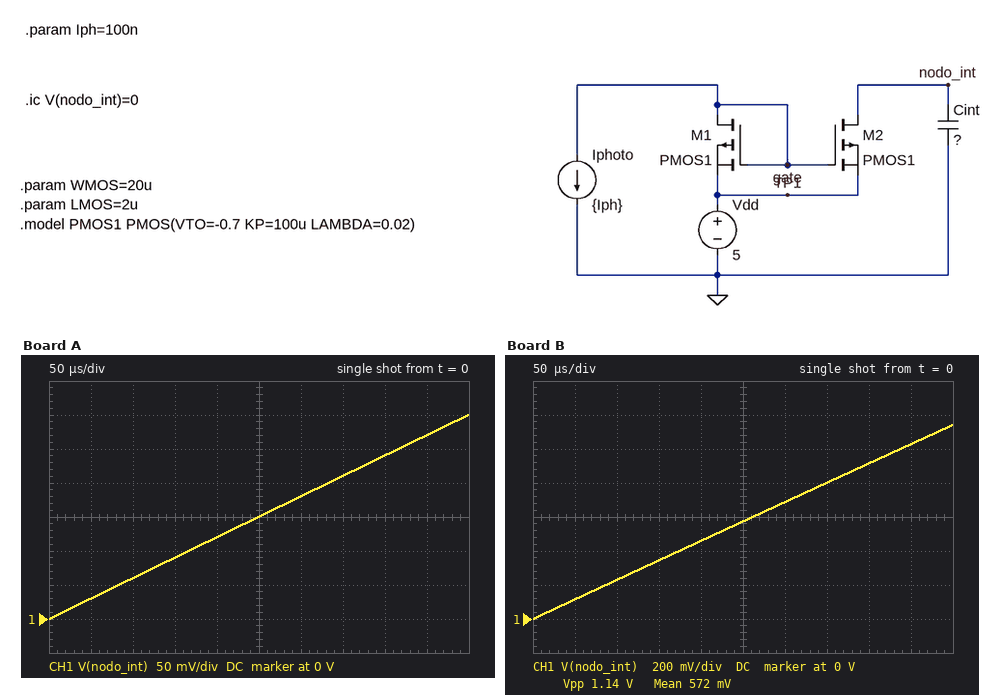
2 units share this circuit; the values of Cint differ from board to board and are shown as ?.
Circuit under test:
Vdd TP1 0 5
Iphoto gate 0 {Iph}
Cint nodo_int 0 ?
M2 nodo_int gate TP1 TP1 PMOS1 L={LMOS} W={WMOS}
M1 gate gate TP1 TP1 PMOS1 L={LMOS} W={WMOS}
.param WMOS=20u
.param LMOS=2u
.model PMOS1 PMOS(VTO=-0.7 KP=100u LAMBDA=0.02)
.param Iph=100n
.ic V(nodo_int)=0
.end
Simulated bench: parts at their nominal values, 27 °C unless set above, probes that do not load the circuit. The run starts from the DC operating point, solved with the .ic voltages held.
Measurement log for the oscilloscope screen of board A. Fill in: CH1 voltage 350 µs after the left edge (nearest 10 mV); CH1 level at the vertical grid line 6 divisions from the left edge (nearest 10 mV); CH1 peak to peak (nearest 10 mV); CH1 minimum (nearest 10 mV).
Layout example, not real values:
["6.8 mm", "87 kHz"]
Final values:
["210 mV", "180 mV", "300 mV", "0 V"]
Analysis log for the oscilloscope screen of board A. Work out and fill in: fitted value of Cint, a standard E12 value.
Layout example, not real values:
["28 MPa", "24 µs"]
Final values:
["180 pF"]
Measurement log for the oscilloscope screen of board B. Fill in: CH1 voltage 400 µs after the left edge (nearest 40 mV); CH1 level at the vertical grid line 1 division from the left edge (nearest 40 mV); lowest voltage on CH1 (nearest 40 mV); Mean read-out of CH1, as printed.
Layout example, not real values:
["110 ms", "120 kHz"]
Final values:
["920 mV", "120 mV", "0 V", "572 mV"]
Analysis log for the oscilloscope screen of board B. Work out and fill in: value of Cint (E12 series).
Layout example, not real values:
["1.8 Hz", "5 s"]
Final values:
["47 pF"]
